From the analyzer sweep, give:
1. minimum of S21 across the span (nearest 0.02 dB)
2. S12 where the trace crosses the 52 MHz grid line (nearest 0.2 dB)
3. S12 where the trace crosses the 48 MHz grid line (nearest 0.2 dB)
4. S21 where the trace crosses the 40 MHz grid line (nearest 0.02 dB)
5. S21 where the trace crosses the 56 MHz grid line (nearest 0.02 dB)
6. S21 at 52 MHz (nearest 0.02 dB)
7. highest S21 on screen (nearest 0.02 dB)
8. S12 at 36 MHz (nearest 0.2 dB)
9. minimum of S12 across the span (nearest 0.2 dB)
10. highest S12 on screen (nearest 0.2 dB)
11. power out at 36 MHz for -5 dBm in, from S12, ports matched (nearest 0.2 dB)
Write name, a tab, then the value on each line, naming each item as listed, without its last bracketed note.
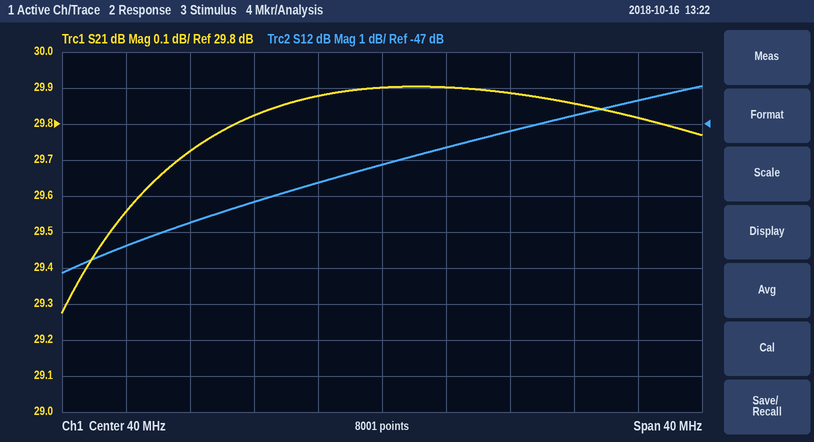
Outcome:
minimum of S21 across the span	29.28 dB
S12 where the trace crosses the 52 MHz grid line	-46.8 dB
S12 where the trace crosses the 48 MHz grid line	-47.2 dB
S21 where the trace crosses the 40 MHz grid line	29.90 dB
S21 where the trace crosses the 56 MHz grid line	29.82 dB
S21 at 52 MHz	29.86 dB
highest S21 on screen	29.90 dB
S12 at 36 MHz	-48.6 dB
minimum of S12 across the span	-51.2 dB
highest S12 on screen	-46.0 dB
power out at 36 MHz for -5 dBm in, from S12, ports matched	-53.6 dBm
